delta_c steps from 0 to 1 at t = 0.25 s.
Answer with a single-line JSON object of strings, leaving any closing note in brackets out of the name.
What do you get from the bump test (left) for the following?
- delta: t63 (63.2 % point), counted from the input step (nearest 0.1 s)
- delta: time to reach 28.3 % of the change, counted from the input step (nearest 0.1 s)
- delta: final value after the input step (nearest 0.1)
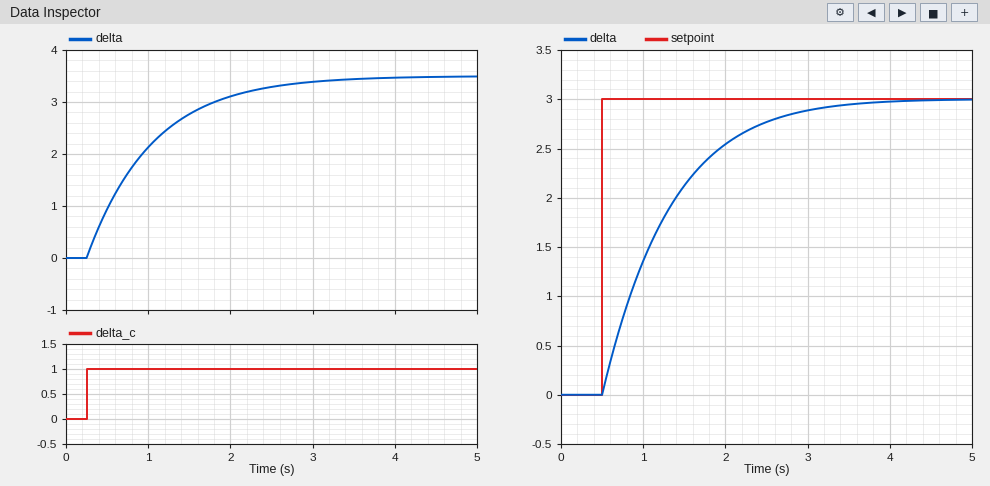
{"delta: t63 (63.2 % point), counted from the input step": "0.8 s", "delta: time to reach 28.3 % of the change, counted from the input step": "0.3 s", "delta: final value after the input step": "3.5"}
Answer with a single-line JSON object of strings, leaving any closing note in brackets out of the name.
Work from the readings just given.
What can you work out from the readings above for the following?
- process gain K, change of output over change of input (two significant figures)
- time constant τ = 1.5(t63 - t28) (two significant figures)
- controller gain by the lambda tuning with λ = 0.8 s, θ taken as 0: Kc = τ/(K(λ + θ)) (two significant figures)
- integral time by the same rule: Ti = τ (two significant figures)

{"process gain K, change of output over change of input": "3.5", "time constant τ = 1.5(t63 - t28)": "0.75 s", "controller gain by the lambda tuning with λ = 0.8 s, θ taken as 0: Kc = τ/(K(λ + θ))": "0.27", "integral time by the same rule: Ti = τ": "0.75 s"}
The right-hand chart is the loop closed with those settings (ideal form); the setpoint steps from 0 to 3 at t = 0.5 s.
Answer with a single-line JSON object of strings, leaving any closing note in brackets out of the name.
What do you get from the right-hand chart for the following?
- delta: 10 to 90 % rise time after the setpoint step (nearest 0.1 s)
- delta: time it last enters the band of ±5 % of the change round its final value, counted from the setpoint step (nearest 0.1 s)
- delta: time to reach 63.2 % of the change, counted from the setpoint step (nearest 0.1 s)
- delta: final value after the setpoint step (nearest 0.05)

{"delta: 10 to 90 % rise time after the setpoint step": "1.7 s", "delta: time it last enters the band of ±5 % of the change round its final value, counted from the setpoint step": "2.3 s", "delta: time to reach 63.2 % of the change, counted from the setpoint step": "0.8 s", "delta: final value after the setpoint step": "3.00"}
